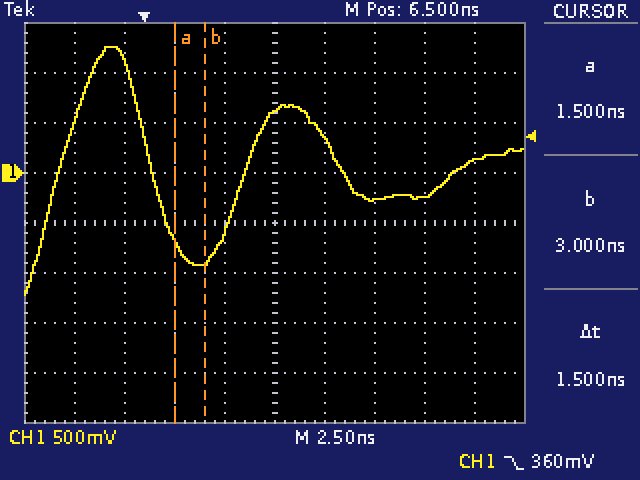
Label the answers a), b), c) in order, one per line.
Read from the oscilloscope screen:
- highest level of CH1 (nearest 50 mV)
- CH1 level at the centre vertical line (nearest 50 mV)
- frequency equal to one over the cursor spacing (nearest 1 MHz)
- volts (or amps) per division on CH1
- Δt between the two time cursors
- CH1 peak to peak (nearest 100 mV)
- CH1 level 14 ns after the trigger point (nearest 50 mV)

a) 1.25 V
b) 600 mV
c) 667 MHz
d) 500 mV
e) 1.5 ns
f) 2.50 V
g) -250 mV
